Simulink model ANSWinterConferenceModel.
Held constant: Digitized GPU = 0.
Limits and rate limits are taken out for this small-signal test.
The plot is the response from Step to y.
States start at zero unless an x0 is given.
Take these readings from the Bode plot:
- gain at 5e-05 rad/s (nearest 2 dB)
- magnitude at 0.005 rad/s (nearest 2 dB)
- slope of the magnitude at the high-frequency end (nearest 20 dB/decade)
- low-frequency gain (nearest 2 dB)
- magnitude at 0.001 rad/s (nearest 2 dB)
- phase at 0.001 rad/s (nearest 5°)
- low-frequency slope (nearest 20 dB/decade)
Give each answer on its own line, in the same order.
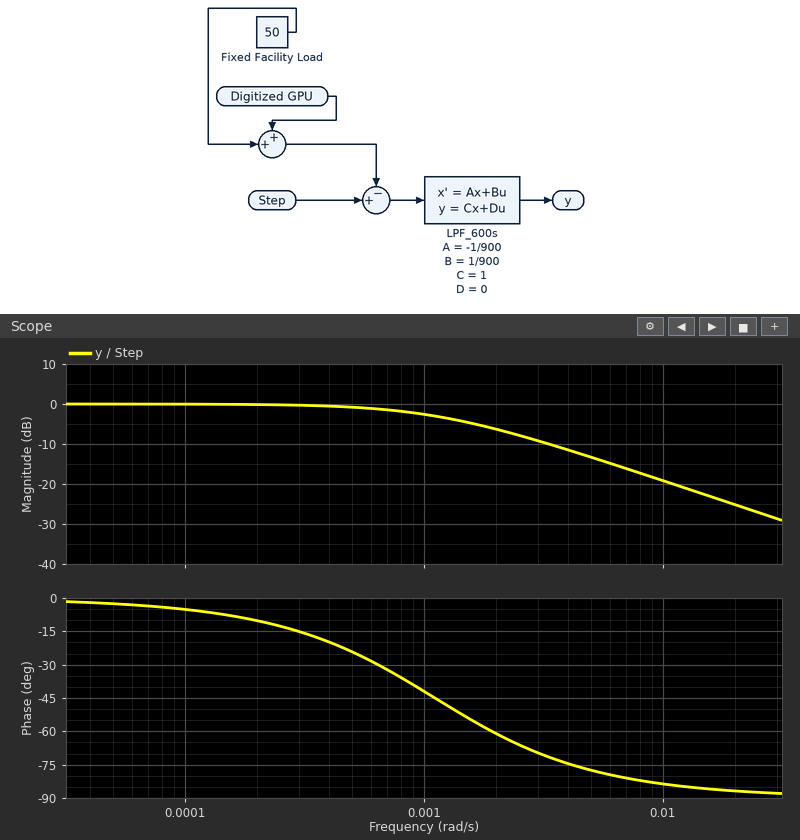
0 dB
-14 dB
-20 dB/decade
0 dB
-2 dB
-40°
0 dB/decade
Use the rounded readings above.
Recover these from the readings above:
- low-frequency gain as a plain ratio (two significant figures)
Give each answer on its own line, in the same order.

1.0
